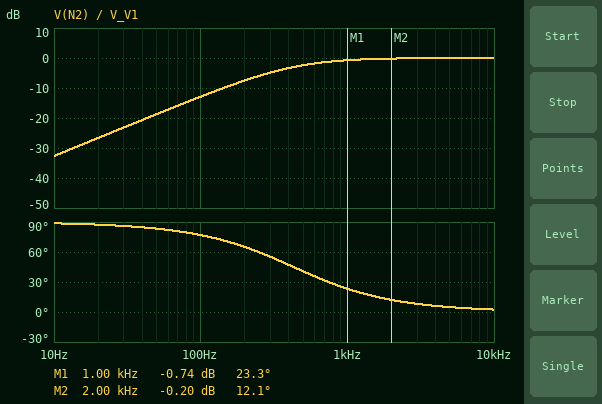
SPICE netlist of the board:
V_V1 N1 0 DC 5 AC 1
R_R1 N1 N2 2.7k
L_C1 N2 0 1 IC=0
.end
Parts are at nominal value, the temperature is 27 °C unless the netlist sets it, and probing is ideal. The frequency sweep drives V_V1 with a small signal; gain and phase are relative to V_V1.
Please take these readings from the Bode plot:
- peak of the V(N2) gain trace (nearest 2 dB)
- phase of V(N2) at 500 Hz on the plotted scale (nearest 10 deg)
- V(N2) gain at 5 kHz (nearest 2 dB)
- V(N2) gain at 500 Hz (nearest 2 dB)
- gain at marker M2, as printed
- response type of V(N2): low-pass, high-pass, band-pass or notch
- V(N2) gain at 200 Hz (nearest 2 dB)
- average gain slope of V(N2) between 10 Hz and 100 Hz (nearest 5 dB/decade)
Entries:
0 dB
40 deg
0 dB
-2 dB
-0.20 dB
high-pass
-8 dB
20 dB/decade
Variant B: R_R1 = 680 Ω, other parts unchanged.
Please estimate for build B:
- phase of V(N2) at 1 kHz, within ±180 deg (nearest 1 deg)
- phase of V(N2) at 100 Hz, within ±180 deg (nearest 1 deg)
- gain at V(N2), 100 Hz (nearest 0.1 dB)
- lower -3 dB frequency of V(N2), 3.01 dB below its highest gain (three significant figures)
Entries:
6 deg
47 deg
-3.4 dB
108 Hz
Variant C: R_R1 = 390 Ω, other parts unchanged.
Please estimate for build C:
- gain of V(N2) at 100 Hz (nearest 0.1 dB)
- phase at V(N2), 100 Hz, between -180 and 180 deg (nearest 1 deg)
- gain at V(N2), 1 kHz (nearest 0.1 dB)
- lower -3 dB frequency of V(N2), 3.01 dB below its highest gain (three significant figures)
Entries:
-1.4 dB
32 deg
0 dB
62.1 Hz
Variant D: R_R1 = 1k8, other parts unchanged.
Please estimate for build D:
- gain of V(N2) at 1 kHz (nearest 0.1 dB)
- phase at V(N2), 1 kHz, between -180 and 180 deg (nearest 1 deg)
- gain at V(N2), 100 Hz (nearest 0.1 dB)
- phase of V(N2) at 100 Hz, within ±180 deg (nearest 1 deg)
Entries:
-0.3 dB
16 deg
-9.6 dB
71 deg
